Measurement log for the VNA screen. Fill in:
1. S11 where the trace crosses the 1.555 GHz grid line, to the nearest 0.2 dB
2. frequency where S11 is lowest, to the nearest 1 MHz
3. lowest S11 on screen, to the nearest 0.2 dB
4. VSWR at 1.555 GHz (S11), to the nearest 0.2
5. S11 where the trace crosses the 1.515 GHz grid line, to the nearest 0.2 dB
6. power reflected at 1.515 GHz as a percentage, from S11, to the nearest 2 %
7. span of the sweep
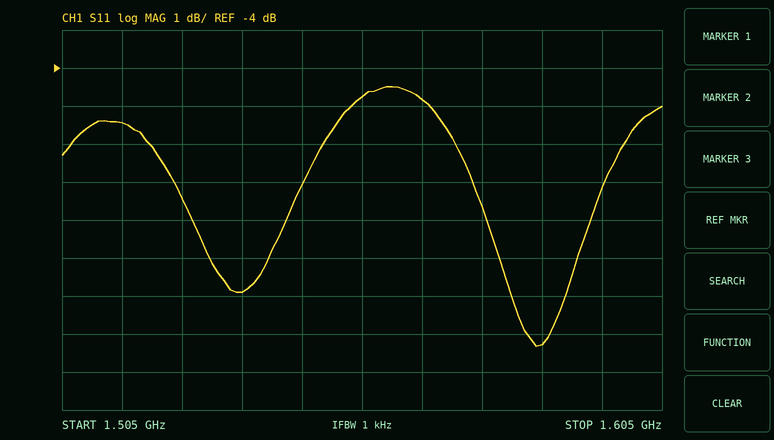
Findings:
-4.8 dB
1.584 GHz
-11.4 dB
3.8
-5.4 dB
28 %
100 MHz
